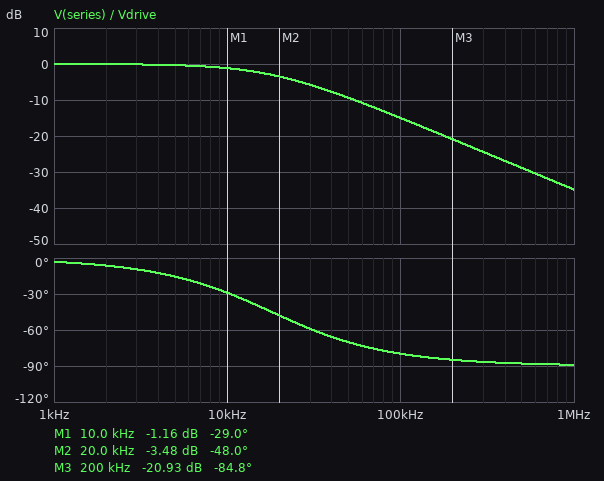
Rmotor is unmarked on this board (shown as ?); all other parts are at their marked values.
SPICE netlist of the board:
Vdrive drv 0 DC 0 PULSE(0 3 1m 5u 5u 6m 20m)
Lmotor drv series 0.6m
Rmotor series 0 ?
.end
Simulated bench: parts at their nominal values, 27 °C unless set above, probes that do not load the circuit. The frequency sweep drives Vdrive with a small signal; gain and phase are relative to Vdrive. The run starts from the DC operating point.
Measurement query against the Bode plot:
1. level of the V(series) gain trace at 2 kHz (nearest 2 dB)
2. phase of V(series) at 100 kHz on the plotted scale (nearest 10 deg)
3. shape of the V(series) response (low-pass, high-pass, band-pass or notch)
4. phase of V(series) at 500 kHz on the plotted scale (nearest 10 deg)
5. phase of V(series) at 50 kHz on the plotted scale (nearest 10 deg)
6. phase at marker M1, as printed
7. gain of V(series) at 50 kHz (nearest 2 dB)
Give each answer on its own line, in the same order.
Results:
0 dB
-80 deg
low-pass
-90 deg
-70 deg
-29.0 deg
-10 dB
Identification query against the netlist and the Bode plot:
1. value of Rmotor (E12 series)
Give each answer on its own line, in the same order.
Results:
68 Ω
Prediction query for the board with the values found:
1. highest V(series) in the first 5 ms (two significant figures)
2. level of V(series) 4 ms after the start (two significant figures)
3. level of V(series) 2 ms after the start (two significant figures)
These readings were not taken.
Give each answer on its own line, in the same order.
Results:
3.0 V
3.0 V
3.0 V
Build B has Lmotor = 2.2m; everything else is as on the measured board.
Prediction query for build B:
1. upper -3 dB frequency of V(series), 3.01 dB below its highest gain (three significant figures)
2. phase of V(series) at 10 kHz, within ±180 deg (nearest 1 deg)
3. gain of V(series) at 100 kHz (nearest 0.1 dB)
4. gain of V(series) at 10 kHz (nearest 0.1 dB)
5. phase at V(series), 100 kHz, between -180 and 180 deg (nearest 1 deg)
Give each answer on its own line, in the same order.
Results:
4.92 kHz
-64 deg
-26.2 dB
-7.1 dB
-87 deg
